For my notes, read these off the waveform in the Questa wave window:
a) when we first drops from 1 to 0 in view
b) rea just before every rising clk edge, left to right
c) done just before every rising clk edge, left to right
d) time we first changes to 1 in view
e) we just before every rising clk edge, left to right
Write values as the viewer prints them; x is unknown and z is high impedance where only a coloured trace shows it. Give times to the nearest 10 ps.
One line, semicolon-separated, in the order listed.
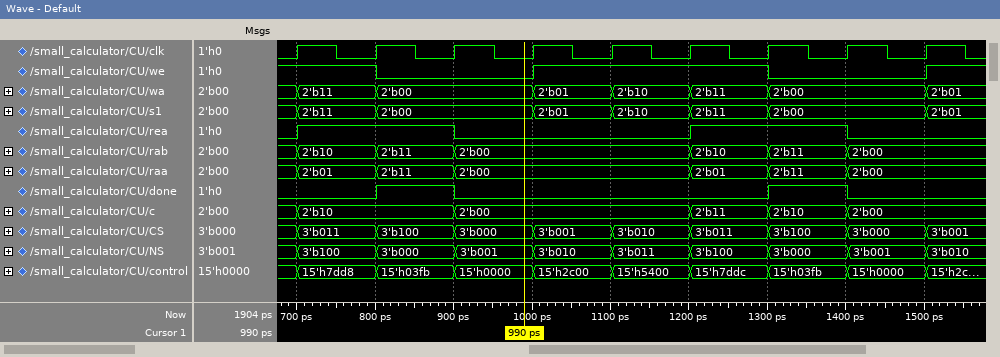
800 ps; 0 1 1 0 0 0 1 1 0; 0 0 1 0 0 0 0 1 0; 1000 ps; 1 1 0 0 1 1 1 0 0
